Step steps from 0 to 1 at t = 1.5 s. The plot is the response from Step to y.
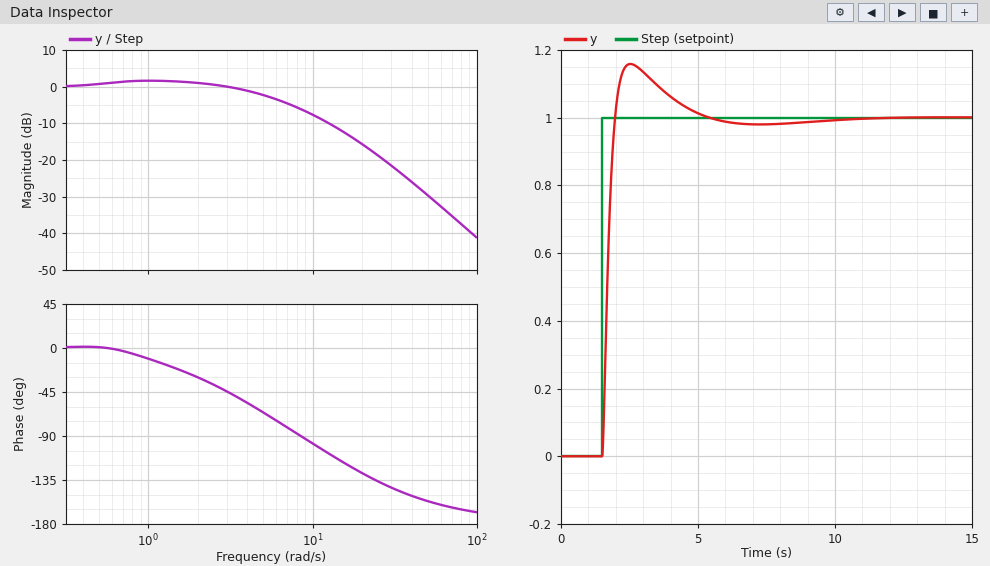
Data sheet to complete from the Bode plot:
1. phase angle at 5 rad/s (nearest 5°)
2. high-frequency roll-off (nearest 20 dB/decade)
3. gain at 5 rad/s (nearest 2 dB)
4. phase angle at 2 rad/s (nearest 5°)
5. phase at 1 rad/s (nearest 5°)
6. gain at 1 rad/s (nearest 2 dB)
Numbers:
-65°
-40 dB/decade
-2 dB
-30°
-10°
2 dB
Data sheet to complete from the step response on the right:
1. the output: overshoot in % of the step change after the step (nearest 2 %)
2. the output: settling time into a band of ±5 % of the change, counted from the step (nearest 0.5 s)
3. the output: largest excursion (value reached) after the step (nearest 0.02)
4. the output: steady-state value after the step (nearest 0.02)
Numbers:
16 %
2.5 s
1.16
1.00
